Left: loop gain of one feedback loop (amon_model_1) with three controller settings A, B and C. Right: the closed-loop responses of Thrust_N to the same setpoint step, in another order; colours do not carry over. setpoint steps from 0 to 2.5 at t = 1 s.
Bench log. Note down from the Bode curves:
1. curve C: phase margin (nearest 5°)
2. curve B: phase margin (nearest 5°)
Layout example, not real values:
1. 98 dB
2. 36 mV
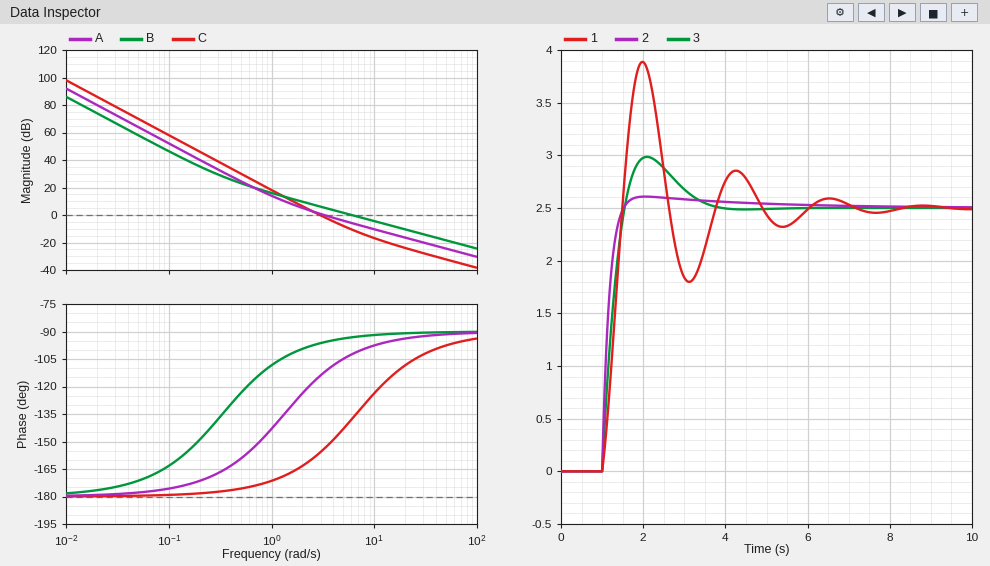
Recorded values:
1. 25°
2. 85°
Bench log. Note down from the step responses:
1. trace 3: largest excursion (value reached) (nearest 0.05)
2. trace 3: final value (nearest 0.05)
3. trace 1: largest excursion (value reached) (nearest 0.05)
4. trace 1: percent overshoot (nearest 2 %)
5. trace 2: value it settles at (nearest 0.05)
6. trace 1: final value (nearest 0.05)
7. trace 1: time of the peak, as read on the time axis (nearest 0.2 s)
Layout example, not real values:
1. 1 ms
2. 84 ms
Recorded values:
1. 3.00
2. 2.50
3. 3.90
4. 56 %
5. 2.50
6. 2.50
7. 2.0 s
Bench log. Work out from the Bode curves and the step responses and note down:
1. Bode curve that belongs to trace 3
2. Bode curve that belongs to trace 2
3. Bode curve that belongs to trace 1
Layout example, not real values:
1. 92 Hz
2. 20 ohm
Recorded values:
1. A
2. B
3. C
